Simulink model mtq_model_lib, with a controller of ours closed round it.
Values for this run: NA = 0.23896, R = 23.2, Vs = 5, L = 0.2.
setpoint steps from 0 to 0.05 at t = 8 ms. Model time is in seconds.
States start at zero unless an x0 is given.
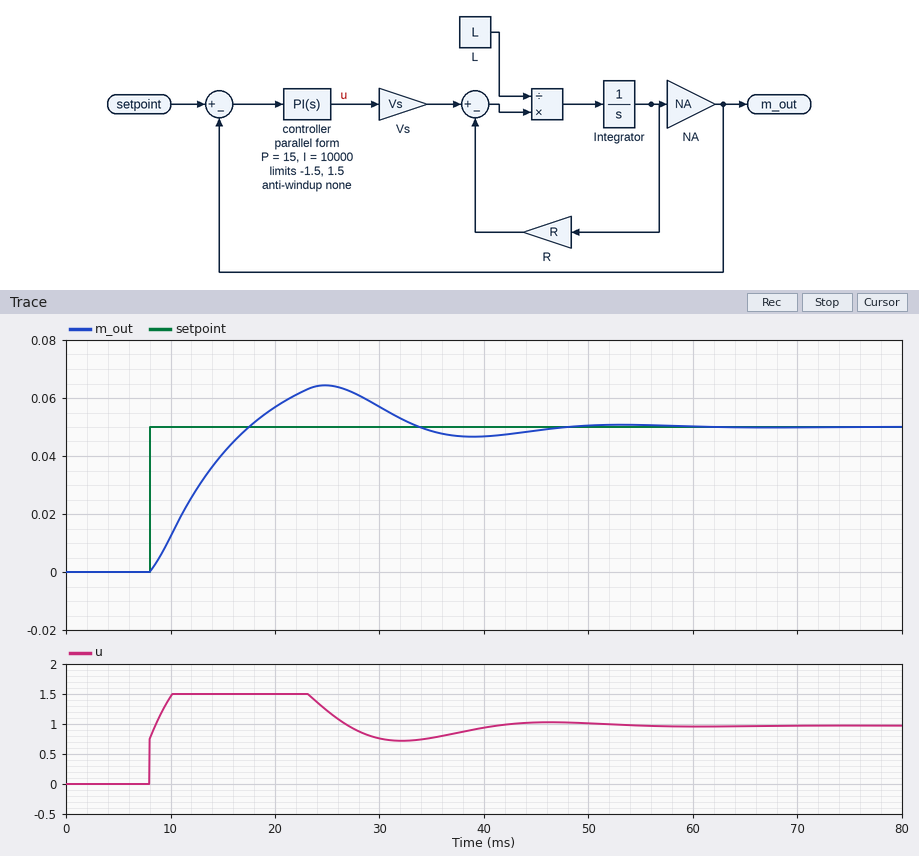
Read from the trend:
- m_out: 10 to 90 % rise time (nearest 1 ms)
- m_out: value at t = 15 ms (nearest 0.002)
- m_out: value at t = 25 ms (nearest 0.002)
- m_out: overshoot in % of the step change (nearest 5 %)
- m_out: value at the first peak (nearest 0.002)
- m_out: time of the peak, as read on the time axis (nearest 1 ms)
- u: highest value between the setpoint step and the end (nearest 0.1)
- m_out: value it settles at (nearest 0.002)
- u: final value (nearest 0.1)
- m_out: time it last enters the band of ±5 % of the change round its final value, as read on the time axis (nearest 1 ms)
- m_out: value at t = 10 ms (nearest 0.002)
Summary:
7 ms
0.040
0.064
30 %
0.064
25 ms
1.5
0.050
1.0
42 ms
0.012
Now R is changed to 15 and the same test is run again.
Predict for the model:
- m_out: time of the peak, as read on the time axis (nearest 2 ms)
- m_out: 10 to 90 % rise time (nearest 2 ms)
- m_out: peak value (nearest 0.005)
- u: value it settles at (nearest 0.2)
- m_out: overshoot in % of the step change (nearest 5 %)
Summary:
22 ms
6 ms
0.070
0.6
40 %
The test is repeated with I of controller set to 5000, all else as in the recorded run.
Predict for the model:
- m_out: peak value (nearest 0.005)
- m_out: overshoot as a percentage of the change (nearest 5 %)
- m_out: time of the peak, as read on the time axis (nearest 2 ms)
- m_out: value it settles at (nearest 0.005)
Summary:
0.055
10 %
26 ms
0.050
